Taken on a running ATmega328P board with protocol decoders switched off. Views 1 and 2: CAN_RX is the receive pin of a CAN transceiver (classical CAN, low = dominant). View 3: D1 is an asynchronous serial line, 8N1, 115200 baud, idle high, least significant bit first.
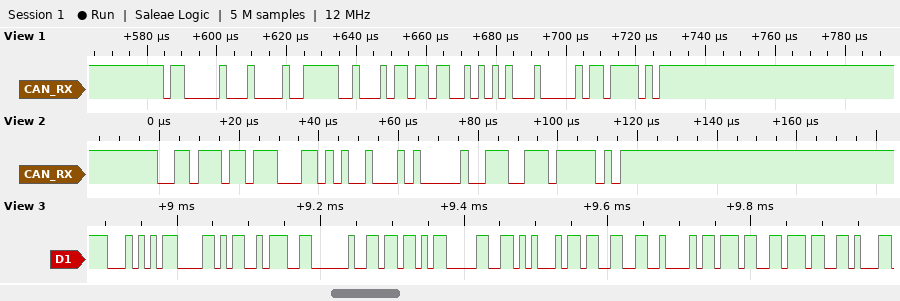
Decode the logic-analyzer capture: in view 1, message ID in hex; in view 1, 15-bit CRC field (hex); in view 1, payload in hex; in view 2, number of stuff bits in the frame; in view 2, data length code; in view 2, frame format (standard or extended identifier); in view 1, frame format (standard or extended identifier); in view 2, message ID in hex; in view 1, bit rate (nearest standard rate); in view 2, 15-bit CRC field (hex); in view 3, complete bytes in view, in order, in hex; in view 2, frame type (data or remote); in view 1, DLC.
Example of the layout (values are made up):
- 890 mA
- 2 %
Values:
- 0x601
- 0x40DE
- FA 2D B2 A8
- 2
- 0
- extended
- standard
- 0x0DDA3522
- 500 kbit/s
- 0x39DF
- 54 58 3A 20 5B 30 45 33 42 37 37
- remote
- 4
